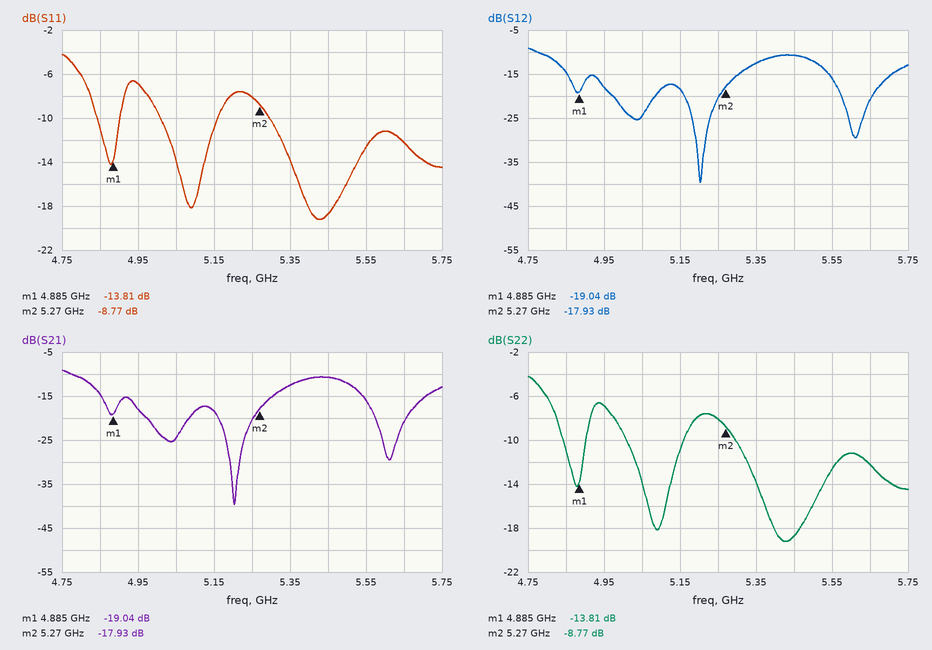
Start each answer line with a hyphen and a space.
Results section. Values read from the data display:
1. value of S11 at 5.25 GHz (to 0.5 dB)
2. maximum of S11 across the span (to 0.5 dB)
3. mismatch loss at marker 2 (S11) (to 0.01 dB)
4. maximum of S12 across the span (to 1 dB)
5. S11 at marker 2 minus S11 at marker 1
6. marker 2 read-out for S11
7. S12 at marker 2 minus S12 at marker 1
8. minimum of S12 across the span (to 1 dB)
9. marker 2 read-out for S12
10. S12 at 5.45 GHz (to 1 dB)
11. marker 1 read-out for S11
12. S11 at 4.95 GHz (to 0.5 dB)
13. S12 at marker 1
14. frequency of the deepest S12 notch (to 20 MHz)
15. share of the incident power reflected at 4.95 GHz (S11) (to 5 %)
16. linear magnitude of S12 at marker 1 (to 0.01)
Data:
- -8.0 dB
- -4.0 dB
- 0.62 dB
- -9 dB
- 5.04 dB
- -8.77 dB
- 1.11 dB
- -40 dB
- -17.93 dB
- -11 dB
- -13.81 dB
- -7.0 dB
- -19.04 dB
- 5.20 GHz
- 20 %
- 0.11
